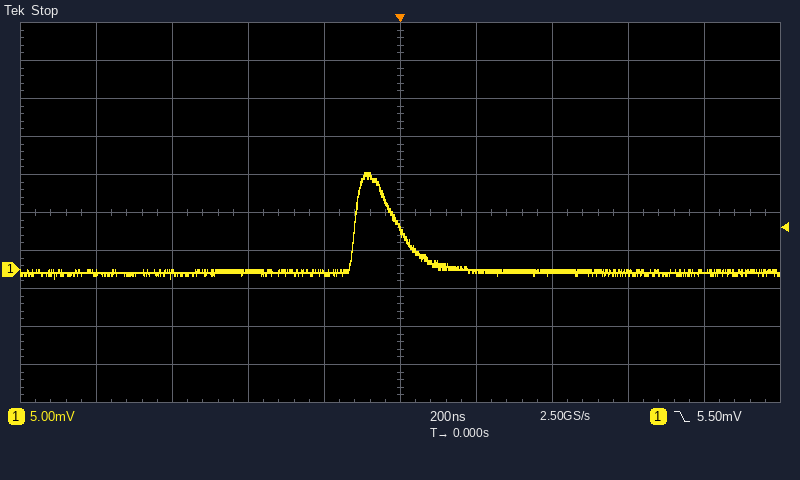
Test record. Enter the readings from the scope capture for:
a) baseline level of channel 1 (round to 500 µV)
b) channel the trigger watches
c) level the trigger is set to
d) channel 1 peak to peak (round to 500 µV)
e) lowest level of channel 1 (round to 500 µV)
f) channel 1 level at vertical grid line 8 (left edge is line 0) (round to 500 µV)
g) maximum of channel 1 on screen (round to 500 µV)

-500 µV
channel 1
5.50 mV
14.0 mV
-1.0 mV
-500 µV
13.0 mV
